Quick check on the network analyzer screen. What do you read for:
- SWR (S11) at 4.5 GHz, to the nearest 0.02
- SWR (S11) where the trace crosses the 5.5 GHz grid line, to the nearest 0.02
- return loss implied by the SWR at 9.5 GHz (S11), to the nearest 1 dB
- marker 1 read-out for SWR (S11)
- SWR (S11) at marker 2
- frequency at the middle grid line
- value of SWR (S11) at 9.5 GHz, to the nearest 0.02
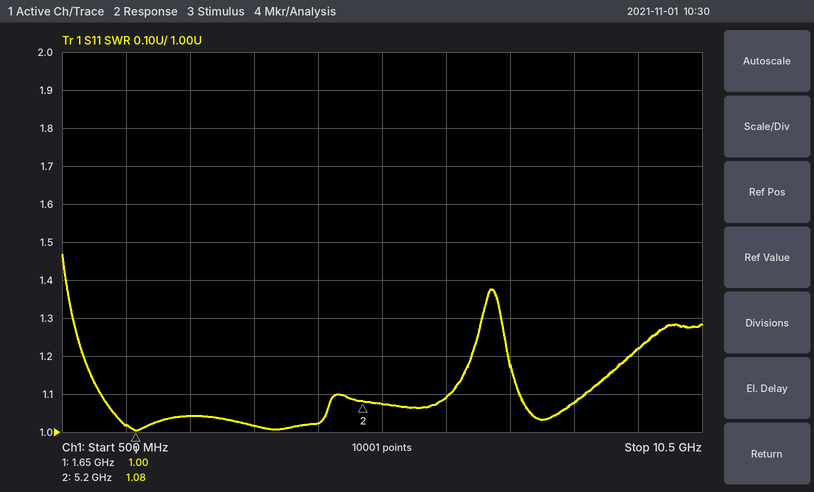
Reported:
1.02
1.08
20 dB
1.00
1.08
5.5 GHz
1.22
